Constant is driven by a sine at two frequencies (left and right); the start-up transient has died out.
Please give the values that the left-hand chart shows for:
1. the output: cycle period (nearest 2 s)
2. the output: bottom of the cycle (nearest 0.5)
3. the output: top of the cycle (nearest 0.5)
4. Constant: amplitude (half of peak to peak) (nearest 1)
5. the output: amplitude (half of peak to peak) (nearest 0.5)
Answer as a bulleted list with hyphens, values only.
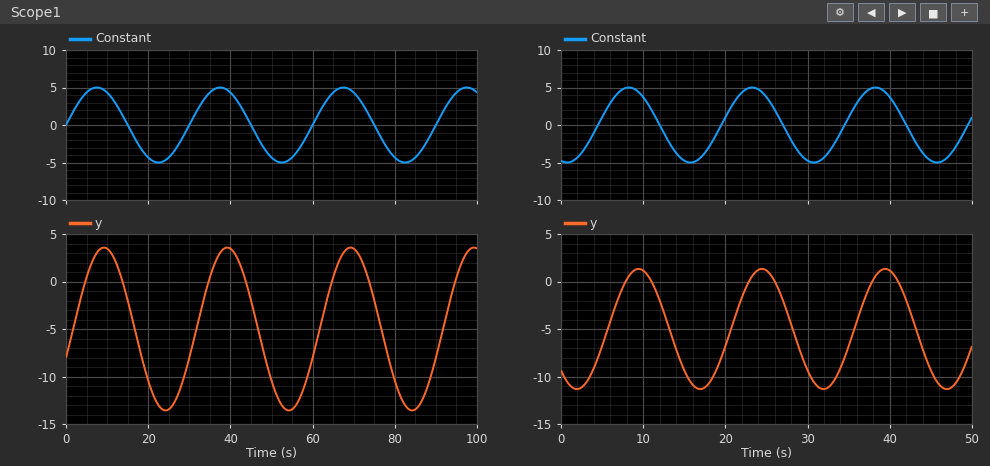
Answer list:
- 30 s
- -13.5
- 3.5
- 5
- 8.5
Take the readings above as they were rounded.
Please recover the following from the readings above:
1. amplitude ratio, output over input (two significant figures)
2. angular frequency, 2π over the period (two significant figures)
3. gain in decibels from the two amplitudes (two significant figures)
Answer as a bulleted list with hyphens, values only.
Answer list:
- 1.7
- 0.21 rad/s
- 4.6 dB
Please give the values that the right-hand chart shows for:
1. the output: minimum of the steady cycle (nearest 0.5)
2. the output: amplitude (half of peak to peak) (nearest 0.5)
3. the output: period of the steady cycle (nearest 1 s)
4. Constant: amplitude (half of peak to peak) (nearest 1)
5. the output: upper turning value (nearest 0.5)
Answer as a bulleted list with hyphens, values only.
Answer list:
- -11.5
- 6.5
- 15 s
- 5
- 1.5
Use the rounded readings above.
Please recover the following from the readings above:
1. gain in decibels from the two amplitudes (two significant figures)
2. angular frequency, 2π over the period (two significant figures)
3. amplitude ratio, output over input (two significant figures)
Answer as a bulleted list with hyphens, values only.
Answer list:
- 2.3 dB
- 0.42 rad/s
- 1.3
